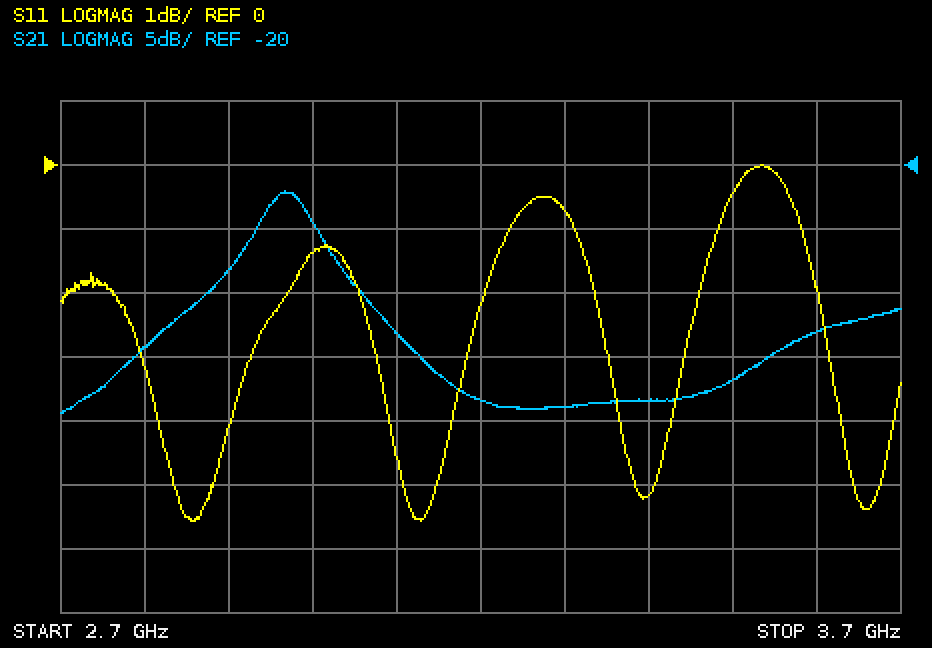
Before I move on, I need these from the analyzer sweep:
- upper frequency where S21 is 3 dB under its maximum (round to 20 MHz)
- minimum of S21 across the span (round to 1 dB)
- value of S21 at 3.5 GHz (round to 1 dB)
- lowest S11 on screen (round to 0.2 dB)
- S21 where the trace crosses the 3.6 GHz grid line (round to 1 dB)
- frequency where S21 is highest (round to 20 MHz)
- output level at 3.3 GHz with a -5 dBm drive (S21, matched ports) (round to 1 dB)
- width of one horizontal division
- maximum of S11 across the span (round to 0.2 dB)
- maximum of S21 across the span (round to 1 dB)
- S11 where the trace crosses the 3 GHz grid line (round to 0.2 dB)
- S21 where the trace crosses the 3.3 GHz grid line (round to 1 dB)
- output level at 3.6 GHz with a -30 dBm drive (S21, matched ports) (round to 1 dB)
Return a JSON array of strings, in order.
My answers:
["3.00 GHz", "-39 dB", "-37 dB", "-5.6 dB", "-33 dB", "2.96 GHz", "-44 dBm", "100 MHz", "0.0 dB", "-22 dB", "-1.4 dB", "-39 dB", "-63 dBm"]
